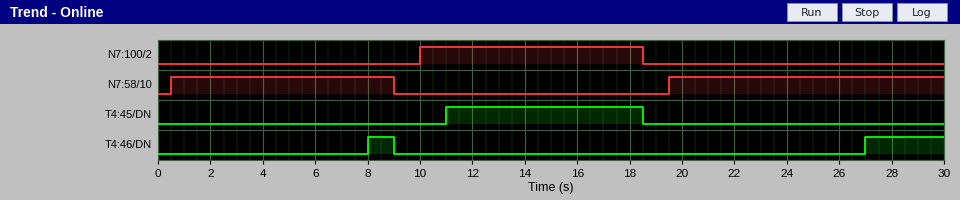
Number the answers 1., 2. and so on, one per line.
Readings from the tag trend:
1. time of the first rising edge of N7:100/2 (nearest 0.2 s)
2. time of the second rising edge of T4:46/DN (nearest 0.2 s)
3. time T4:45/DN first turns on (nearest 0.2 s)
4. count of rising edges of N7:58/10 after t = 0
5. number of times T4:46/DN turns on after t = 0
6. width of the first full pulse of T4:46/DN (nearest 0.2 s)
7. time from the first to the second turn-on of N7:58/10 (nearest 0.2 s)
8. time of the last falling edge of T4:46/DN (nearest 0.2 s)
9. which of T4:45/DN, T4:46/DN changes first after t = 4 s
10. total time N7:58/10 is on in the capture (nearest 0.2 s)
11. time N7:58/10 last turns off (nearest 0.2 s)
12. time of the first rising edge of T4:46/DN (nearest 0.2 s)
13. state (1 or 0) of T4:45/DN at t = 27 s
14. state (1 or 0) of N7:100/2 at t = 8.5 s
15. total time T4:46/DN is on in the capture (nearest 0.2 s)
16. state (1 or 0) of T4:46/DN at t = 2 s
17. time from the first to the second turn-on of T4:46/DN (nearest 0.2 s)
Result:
1. 10.0 s
2. 27.0 s
3. 11.0 s
4. 2
5. 2
6. 1.0 s
7. 19.0 s
8. 9.0 s
9. T4:46/DN
10. 19.0 s
11. 9.0 s
12. 8.0 s
13. 0
14. 0
15. 4.0 s
16. 0
17. 19.0 s
